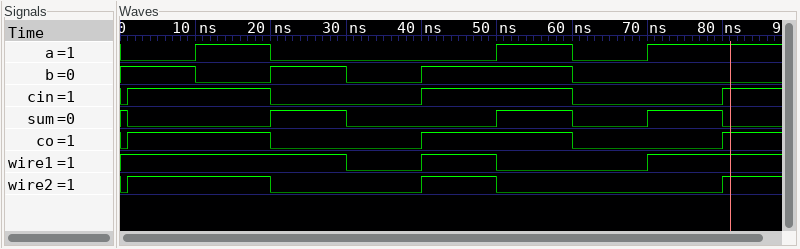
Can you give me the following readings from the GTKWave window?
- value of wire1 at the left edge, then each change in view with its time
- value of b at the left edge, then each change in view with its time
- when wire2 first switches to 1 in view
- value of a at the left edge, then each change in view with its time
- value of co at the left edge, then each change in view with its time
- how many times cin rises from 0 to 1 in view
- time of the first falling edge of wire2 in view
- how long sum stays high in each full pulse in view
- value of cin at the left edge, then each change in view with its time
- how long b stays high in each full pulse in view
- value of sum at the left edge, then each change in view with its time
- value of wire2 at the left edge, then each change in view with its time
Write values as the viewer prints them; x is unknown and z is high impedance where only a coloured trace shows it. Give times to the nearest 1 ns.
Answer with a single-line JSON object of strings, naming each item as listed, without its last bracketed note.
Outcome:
{"value of wire1 at the left edge, then each change in view with its time": "1, 0 at 30 ns, 1 at 40 ns, 0 at 50 ns, 1 at 70 ns", "value of b at the left edge, then each change in view with its time": "1, 0 at 10 ns, 1 at 20 ns, 0 at 30 ns, 1 at 40 ns, 0 at 60 ns", "when wire2 first switches to 1 in view": "1 ns", "value of a at the left edge, then each change in view with its time": "0, 1 at 10 ns, 0 at 20 ns, 1 at 50 ns, 0 at 60 ns, 1 at 70 ns", "value of co at the left edge, then each change in view with its time": "0, 1 at 1 ns, 0 at 20 ns, 1 at 40 ns, 0 at 60 ns, 1 at 80 ns", "how many times cin rises from 0 to 1 in view": "3", "time of the first falling edge of wire2 in view": "20 ns", "how long sum stays high in each full pulse in view": "10 ns, 10 ns, 10 ns", "value of cin at the left edge, then each change in view with its time": "0, 1 at 1 ns, 0 at 20 ns, 1 at 40 ns, 0 at 60 ns, 1 at 80 ns", "how long b stays high in each full pulse in view": "10 ns, 20 ns", "value of sum at the left edge, then each change in view with its time": "1, 0 at 1 ns, 1 at 20 ns, 0 at 30 ns, 1 at 50 ns, 0 at 60 ns, 1 at 70 ns, 0 at 80 ns", "value of wire2 at the left edge, then each change in view with its time": "0, 1 at 1 ns, 0 at 20 ns, 1 at 40 ns, 0 at 50 ns, 1 at 80 ns"}
